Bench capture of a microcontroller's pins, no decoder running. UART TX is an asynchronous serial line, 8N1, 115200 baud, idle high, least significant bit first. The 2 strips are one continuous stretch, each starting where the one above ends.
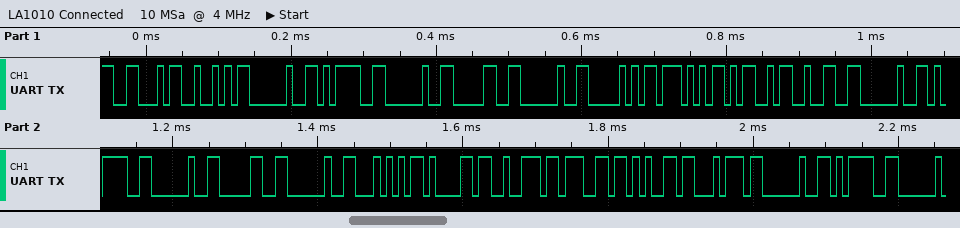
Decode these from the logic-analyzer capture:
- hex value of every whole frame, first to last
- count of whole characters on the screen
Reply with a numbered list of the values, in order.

1. 46 52 20 3D 20 30 20 50 57 4D 32 20 3D 20 30 20 54 61 72 67 65 74 20 3D
2. 24
